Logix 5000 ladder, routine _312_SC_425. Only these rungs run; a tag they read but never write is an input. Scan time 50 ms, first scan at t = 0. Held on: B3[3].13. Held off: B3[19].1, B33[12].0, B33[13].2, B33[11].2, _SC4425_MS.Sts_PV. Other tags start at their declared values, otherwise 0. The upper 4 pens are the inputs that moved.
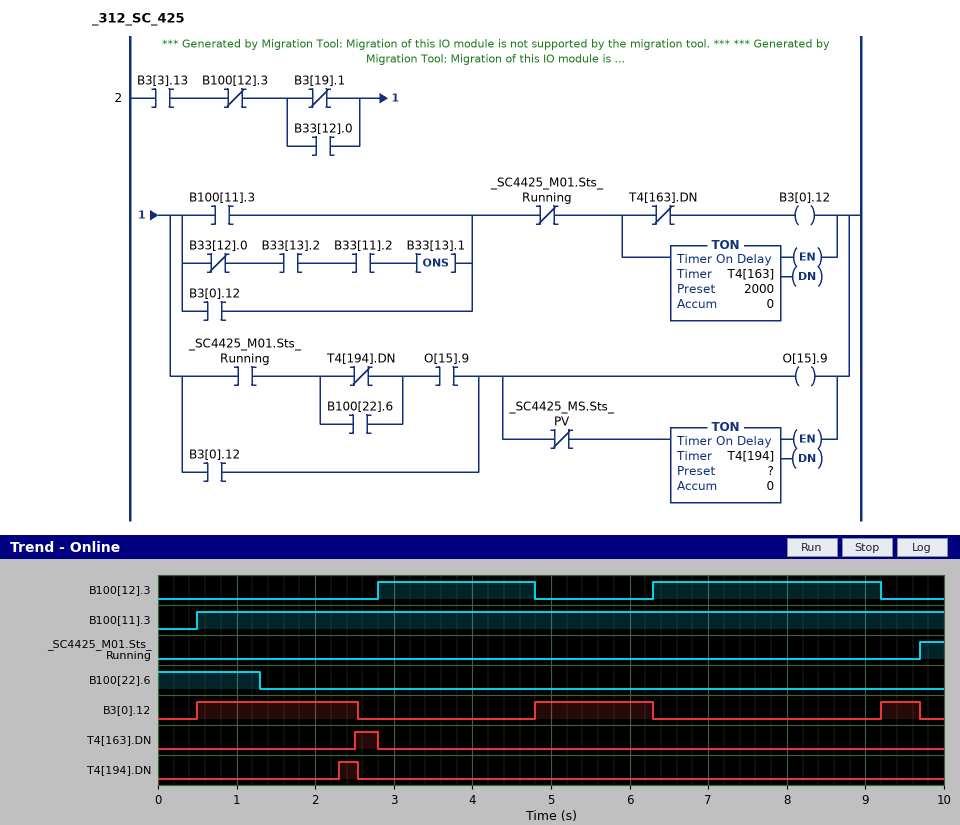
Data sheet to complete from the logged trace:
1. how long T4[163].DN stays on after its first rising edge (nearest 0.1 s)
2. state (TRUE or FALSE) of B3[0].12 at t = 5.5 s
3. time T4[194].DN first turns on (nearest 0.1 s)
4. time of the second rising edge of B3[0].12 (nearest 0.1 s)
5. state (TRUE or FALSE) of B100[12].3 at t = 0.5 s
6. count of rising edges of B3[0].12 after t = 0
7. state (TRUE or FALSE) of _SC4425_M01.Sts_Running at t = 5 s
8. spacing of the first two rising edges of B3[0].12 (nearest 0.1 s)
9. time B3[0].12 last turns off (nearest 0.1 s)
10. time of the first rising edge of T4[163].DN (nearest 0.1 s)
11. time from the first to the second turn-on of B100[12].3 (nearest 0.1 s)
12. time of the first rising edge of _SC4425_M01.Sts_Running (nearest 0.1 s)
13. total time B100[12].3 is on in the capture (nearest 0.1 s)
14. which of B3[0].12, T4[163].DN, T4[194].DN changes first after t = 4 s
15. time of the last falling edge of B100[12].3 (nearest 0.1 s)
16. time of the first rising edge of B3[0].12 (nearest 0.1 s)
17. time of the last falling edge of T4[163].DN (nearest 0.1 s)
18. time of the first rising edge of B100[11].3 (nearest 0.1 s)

0.3 s
TRUE
2.3 s
4.8 s
FALSE
3
FALSE
4.3 s
9.7 s
2.5 s
3.5 s
9.7 s
4.9 s
B3[0].12
9.2 s
0.5 s
2.8 s
0.5 s
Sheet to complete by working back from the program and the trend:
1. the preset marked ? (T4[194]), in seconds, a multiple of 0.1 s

1.8 s
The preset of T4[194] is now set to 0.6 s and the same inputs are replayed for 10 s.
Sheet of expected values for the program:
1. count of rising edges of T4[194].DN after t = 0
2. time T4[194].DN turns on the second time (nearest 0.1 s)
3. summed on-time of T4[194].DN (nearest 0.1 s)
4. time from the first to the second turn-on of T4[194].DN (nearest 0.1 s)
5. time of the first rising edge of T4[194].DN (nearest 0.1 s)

3
5.4 s
2.4 s
4.3 s
1.1 s
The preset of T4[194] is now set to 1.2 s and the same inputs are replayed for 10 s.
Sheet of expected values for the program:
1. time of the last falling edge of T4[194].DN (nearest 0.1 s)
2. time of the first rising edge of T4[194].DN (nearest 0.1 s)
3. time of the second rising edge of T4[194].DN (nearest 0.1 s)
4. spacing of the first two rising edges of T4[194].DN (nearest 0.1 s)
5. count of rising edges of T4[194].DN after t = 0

6.3 s
1.7 s
6.0 s
4.3 s
2
